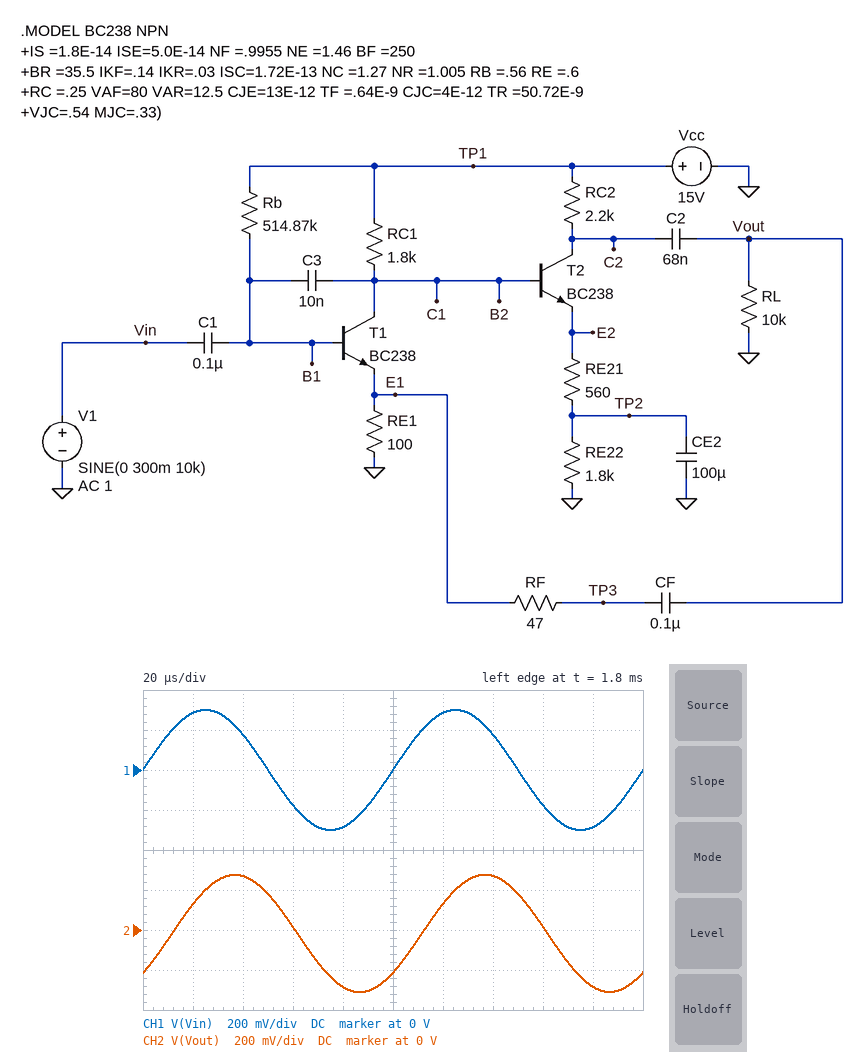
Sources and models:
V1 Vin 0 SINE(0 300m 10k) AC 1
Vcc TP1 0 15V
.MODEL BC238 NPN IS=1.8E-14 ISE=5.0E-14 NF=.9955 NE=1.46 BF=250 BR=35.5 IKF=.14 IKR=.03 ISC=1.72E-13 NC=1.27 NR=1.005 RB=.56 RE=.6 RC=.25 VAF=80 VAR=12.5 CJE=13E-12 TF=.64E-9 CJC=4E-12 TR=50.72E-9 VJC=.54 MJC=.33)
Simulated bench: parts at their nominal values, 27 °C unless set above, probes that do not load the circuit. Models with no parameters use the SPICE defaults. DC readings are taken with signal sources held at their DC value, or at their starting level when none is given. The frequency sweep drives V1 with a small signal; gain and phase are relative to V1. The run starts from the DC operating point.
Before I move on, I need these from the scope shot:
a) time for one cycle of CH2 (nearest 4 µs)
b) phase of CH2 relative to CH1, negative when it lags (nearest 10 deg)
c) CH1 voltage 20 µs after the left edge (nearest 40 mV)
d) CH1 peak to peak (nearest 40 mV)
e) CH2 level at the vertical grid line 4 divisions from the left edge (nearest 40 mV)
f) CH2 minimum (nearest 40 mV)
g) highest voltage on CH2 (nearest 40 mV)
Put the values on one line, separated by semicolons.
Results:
100 µs; -40 deg; 280 mV; 600 mV; -280 mV; -320 mV; 280 mV
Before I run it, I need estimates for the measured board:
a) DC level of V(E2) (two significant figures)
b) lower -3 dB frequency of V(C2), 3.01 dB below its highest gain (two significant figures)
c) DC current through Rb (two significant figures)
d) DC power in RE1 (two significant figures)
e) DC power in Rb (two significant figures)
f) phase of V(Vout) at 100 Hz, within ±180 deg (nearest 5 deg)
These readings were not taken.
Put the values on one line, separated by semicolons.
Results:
4.4 V; 31 Hz; 27 µA; 3.1 mW; 370 µW; 55 deg
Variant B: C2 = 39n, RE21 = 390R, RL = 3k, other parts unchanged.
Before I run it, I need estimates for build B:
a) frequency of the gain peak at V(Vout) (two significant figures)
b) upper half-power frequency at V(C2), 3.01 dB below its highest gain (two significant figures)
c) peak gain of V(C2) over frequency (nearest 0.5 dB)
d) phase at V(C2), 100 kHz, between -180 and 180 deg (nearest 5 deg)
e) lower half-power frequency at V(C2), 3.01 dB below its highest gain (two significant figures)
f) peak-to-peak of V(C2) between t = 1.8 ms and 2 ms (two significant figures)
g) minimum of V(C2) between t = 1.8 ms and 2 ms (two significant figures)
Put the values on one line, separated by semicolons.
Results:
600 Hz; 1.1 kHz; 30.5 dB; -5 deg; 35 Hz; 1.8 V; 9.7 V
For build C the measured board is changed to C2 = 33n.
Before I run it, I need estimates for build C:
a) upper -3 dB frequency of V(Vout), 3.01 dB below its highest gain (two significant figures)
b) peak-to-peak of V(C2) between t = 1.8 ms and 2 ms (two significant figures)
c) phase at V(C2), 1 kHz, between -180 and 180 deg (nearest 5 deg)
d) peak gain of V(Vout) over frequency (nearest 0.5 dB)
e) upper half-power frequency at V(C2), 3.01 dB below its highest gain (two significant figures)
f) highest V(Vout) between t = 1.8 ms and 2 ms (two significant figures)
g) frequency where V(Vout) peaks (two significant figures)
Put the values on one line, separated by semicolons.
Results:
1.5 kHz; 1.7 V; -35 deg; 15.0 dB; 1.3 kHz; 290 mV; 400 Hz
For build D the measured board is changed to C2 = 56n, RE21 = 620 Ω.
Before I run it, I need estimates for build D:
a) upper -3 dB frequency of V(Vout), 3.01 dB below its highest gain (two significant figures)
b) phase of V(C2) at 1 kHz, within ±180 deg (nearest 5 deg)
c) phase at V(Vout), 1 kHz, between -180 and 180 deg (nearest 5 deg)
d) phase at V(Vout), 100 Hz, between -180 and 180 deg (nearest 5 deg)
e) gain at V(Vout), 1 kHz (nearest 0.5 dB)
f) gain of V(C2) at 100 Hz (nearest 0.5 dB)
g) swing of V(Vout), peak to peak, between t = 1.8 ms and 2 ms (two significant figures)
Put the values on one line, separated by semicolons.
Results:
1.1 kHz; -45 deg; -35 deg; 60 deg; 14.5 dB; 26.0 dB; 560 mV
